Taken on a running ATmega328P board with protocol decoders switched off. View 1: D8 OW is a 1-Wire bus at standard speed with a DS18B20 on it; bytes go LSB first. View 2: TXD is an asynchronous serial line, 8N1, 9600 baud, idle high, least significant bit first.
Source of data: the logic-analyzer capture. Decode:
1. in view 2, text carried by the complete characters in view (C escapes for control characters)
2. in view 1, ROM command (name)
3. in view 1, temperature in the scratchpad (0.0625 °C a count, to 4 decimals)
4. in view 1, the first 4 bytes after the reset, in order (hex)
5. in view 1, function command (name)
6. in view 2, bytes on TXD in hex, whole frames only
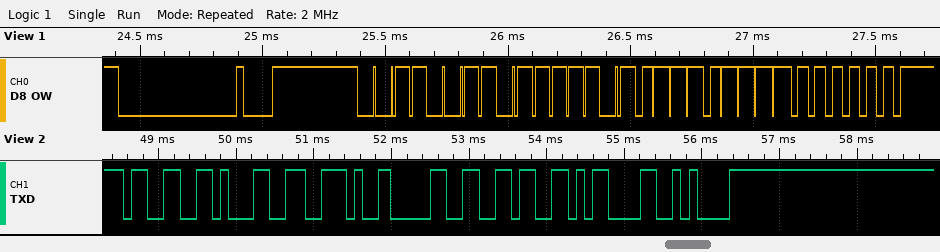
"31.06\r\n"
Skip ROM
30.8750 °C
CC BE EE 01
Read Scratchpad
33 31 2E 30 36 0D 0A
